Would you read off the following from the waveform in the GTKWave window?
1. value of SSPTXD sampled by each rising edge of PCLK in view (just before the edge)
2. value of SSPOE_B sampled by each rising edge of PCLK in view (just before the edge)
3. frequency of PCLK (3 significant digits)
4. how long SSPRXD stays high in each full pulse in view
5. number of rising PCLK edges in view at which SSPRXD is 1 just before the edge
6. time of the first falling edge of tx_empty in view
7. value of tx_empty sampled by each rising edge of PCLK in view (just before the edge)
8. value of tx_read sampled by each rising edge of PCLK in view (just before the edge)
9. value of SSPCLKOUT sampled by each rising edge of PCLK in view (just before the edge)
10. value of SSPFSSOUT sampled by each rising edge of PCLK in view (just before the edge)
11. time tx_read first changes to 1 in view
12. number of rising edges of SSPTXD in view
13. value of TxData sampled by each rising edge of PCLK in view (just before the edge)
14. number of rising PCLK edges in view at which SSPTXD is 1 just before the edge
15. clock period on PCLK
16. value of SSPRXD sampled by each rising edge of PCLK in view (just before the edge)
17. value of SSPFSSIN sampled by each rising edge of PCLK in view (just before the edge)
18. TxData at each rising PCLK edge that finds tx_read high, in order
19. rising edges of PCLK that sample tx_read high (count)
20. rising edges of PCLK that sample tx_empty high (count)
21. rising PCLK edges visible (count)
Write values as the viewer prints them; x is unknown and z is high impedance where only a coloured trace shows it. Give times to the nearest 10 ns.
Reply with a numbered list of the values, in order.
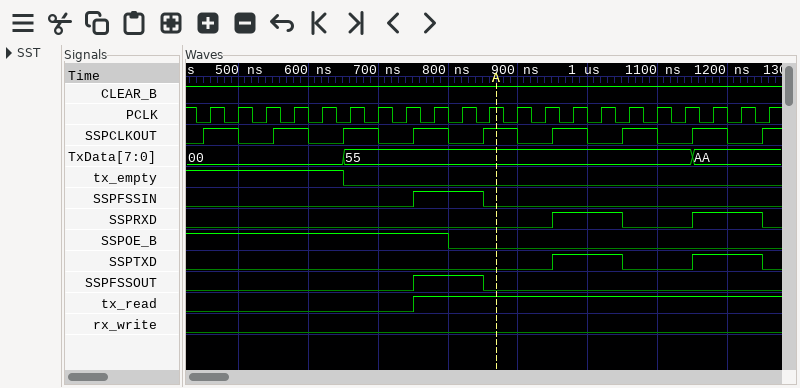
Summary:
1. 0 0 0 0 0 0 0 0 0 0 0 0 0 1 1 0 0 0 1 1 0
2. 1 1 1 1 1 1 1 1 1 0 0 0 0 0 0 0 0 0 0 0 0
3. 25.0 MHz
4. 100 ns, 100 ns
5. 4
6. 650 ns
7. 1 1 1 1 1 0 0 0 0 0 0 0 0 0 0 0 0 0 0 0 0
8. 0 0 0 0 0 0 0 0 1 1 1 1 1 1 1 1 1 1 1 1 1
9. 1 1 0 1 0 1 1 0 1 0 1 1 0 1 0 1 1 0 1 0 1
10. 0 0 0 0 0 0 0 0 1 1 0 0 0 0 0 0 0 0 0 0 0
11. 750 ns
12. 2
13. 00, 00, 00, 00, 00, 55, 55, 55, 55, 55, 55, 55, 55, 55, 55, 55, 55, 55, AA, AA, AA
14. 4
15. 40 ns
16. 0 0 0 0 0 0 0 0 0 0 0 0 0 1 1 0 0 0 1 1 0
17. 0 0 0 0 0 0 0 0 1 1 0 0 0 0 0 0 0 0 0 0 0
18. 55, 55, 55, 55, 55, 55, 55, 55, 55, 55, AA, AA, AA
19. 13
20. 5
21. 21
